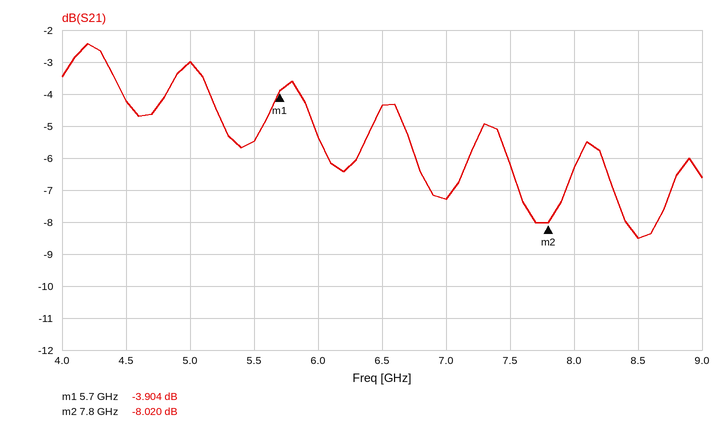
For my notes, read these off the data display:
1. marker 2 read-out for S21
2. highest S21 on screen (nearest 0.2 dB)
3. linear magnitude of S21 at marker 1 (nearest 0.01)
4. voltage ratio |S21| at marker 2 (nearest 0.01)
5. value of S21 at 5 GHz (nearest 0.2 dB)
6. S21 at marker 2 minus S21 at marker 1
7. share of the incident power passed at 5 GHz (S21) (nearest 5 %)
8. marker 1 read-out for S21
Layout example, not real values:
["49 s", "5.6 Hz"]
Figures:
["-8.020 dB", "-2.4 dB", "0.64", "0.40", "-3.0 dB", "-4.116 dB", "50 %", "-3.904 dB"]
